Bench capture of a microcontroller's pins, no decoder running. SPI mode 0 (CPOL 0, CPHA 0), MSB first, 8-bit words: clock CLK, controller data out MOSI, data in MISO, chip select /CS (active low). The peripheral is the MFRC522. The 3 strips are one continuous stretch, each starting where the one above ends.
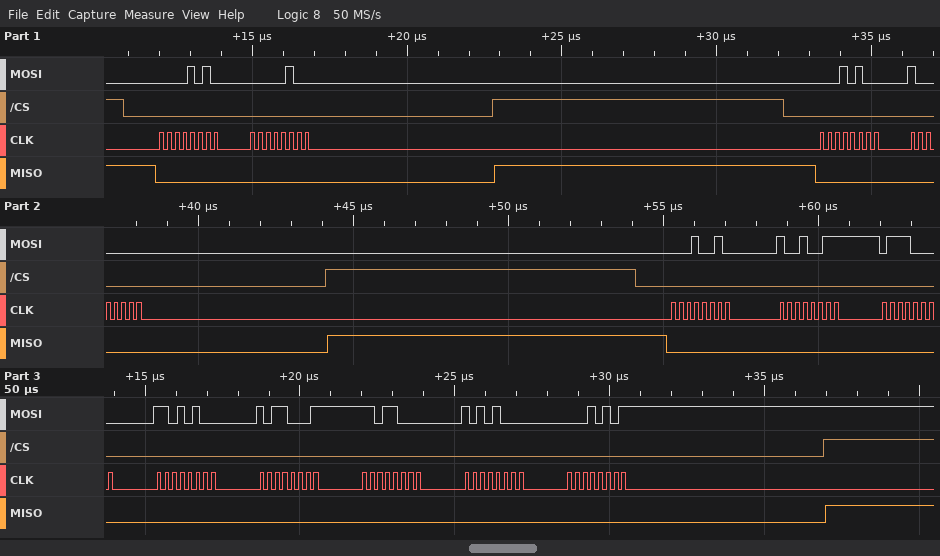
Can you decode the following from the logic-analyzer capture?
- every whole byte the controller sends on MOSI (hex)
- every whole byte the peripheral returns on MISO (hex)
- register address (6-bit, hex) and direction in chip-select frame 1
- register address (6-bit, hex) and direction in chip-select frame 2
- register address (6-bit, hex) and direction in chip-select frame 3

0A 04 14 80 12 93 70 D4 B1 D8 A8 15
00 00 00 00 00 00 00 00 00 00 00 00
0x05 write
0x0A write
0x09 write
